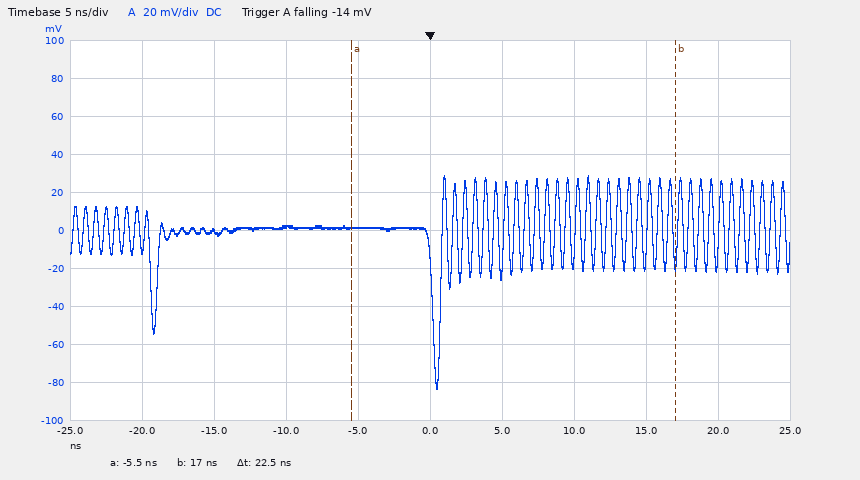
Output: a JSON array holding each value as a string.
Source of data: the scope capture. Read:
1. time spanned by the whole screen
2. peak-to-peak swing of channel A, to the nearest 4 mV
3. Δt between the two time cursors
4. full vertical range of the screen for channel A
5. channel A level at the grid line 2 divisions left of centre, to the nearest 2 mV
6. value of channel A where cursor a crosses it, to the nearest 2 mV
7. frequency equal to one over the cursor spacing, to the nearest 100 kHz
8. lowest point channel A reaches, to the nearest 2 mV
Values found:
["50 ns", "112 mV", "22.5 ns", "200 mV", "2 mV", "2 mV", "44.4 MHz", "-84 mV"]
